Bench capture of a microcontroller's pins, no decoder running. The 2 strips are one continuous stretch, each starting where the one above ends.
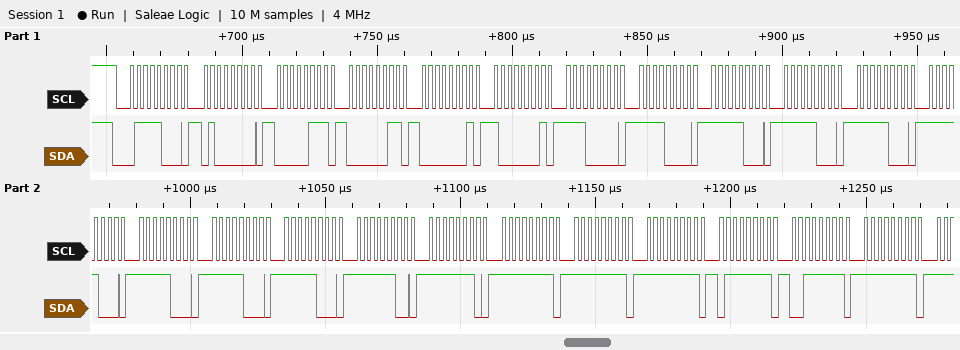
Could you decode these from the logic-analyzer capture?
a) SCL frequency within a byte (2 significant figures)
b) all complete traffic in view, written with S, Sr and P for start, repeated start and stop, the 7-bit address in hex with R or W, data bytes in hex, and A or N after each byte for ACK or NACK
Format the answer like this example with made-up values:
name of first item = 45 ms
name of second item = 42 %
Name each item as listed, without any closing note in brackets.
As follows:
SCL frequency within a byte = 400 kHz
all complete traffic in view, written with S, Sr and P for start, repeated start and stop, the 7-bit address in hex with R or W, data bytes in hex, and A or N after each byte for ACK or NACK = S 3CW A 40 A 07 A 03 A 01 A 81 A E0 A F0 A F8 A F8 A F8 A F8 A F8 A F8 A F8 A FC A FE A FF A FF A FF A 7F A 3F A FF A
